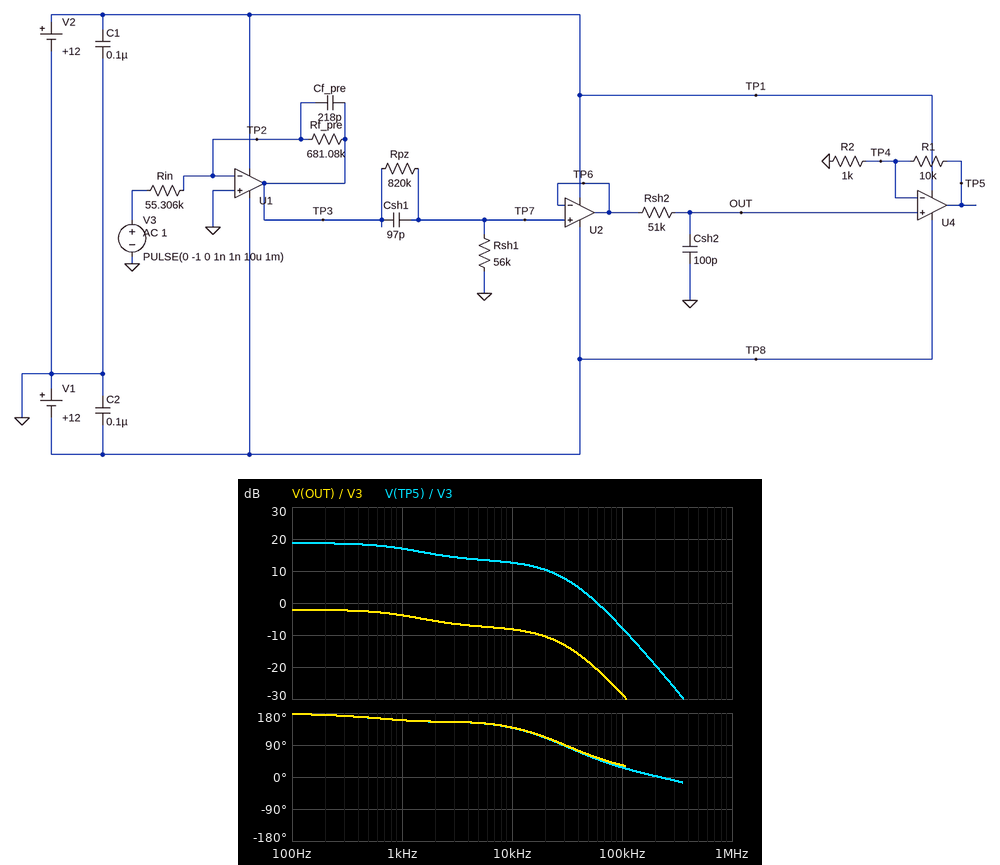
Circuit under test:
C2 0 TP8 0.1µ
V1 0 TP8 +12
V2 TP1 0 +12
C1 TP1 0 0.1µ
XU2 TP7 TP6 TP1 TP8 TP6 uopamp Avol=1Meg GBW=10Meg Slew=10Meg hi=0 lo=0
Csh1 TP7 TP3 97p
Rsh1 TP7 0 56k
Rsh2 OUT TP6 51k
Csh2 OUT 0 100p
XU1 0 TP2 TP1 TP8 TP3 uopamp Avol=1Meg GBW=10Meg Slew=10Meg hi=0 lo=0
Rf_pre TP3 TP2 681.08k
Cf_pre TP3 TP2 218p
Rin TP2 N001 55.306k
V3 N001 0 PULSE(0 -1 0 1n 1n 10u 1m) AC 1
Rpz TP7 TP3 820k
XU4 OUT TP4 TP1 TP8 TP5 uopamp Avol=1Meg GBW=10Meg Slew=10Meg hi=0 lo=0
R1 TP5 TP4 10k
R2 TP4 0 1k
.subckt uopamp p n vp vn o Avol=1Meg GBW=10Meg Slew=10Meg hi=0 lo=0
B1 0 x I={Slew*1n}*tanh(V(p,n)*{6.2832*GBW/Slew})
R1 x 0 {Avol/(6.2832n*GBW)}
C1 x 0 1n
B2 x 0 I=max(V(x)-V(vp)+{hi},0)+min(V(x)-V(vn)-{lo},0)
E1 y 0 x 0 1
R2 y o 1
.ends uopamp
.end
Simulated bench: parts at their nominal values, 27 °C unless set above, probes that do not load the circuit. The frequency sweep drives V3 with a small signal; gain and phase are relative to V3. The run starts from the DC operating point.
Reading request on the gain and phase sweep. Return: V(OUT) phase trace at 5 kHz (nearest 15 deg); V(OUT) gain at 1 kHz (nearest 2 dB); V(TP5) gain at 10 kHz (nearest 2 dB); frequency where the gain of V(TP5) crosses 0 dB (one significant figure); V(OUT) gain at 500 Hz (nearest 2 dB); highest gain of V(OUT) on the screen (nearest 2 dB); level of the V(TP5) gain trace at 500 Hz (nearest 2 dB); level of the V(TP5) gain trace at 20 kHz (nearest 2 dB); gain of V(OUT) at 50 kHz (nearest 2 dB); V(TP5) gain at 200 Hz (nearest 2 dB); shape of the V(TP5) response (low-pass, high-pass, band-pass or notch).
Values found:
150 deg
-4 dB
12 dB
60 kHz
-2 dB
-2 dB
18 dB
10 dB
-18 dB
18 dB
low-pass
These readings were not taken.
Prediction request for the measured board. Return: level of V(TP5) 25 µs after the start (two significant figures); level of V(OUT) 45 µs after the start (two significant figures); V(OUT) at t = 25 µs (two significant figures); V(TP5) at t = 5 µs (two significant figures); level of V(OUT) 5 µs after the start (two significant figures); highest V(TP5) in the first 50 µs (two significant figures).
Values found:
1.0 V
23 mV
90 mV
1.1 V
110 mV
3.0 V
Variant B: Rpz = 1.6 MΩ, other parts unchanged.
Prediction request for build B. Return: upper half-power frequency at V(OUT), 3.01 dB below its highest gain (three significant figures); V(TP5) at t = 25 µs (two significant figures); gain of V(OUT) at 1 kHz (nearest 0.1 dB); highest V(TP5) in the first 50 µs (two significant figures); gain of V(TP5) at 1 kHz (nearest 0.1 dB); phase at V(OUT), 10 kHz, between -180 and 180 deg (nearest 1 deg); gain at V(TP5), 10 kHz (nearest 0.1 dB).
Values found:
20.2 kHz
820 mV
-7.4 dB
2.9 V
13.4 dB
144 deg
12.7 dB
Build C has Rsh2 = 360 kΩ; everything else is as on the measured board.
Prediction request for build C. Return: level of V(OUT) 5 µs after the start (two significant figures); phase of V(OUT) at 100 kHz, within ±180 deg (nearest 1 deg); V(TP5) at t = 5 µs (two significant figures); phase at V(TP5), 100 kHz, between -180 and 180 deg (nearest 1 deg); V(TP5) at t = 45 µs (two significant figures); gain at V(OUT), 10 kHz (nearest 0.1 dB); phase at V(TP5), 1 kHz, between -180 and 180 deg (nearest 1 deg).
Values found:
20 mV
18 deg
210 mV
12 deg
640 mV
-15.7 dB
149 deg
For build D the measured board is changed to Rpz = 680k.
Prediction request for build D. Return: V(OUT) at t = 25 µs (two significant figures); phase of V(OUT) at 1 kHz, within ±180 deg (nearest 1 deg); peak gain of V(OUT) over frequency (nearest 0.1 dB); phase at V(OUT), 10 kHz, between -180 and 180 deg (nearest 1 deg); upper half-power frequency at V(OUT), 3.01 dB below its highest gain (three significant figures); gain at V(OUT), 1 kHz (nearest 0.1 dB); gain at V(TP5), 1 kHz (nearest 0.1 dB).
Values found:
97 mV
156 deg
-0.6 dB
137 deg
1.37 kHz
-2.6 dB
18.2 dB
